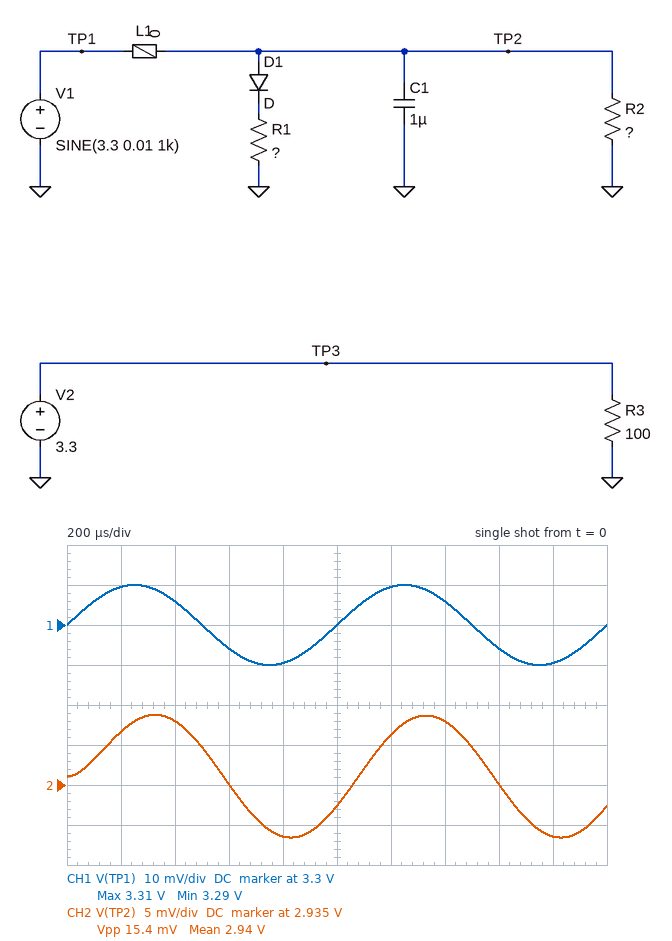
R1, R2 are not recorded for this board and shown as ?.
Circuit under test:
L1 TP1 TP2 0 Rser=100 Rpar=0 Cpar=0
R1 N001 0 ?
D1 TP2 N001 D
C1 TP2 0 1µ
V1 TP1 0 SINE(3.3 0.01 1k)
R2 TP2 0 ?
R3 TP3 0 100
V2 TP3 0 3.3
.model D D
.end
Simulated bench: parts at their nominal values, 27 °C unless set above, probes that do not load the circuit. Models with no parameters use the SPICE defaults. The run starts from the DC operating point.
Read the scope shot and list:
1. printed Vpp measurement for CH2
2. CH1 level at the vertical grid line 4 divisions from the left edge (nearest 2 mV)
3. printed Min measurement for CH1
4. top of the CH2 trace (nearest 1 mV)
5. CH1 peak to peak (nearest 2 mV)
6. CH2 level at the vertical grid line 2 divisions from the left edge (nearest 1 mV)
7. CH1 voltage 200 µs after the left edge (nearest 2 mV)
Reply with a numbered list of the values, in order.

1. 15.4 mV
2. 3.290 V
3. 3.29 V
4. 2.944 V
5. 20 mV
6. 2.943 V
7. 3.310 V
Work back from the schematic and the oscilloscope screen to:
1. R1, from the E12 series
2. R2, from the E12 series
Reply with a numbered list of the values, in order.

1. 820 Ω
2. 3.3 kΩ
